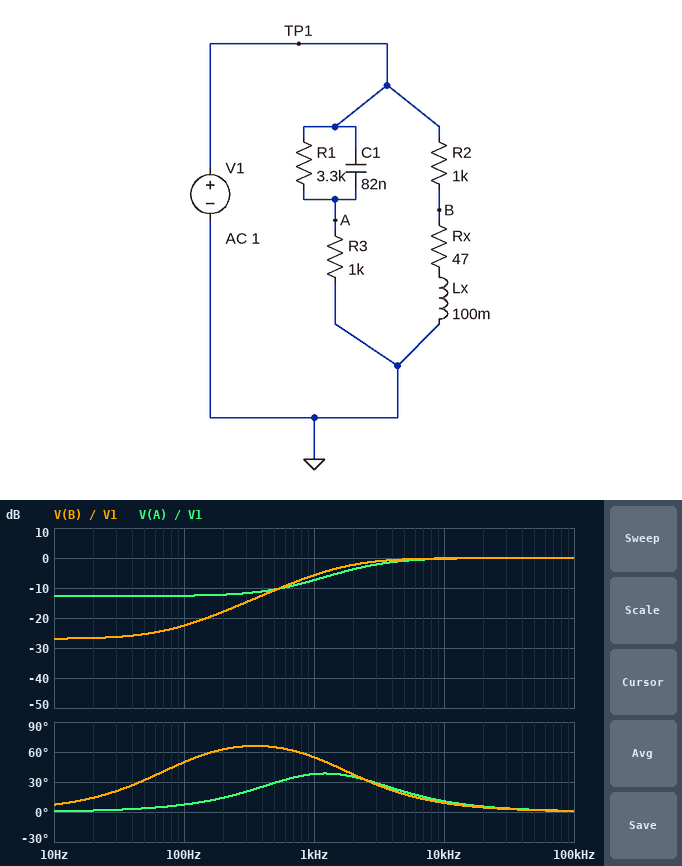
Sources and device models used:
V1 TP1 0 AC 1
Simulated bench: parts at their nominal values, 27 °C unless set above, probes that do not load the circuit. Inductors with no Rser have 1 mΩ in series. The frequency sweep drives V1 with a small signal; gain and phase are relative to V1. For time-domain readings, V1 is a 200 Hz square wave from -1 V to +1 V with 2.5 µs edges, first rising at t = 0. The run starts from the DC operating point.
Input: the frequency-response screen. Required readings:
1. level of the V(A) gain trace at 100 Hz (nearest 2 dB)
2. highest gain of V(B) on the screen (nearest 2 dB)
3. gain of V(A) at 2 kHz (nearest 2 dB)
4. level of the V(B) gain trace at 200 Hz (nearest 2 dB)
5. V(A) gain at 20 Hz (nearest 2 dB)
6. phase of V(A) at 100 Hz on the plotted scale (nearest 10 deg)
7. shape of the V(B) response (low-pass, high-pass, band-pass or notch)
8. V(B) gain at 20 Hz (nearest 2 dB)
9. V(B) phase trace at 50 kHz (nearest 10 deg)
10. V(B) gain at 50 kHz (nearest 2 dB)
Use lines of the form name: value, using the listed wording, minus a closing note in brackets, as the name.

level of the V(A) gain trace at 100 Hz: -12 dB
highest gain of V(B) on the screen: 0 dB
gain of V(A) at 2 kHz: -4 dB
level of the V(B) gain trace at 200 Hz: -18 dB
V(A) gain at 20 Hz: -12 dB
phase of V(A) at 100 Hz on the plotted scale: 10 deg
shape of the V(B) response: high-pass
V(B) gain at 20 Hz: -26 dB
V(B) phase trace at 50 kHz: 0 deg
V(B) gain at 50 kHz: 0 dB
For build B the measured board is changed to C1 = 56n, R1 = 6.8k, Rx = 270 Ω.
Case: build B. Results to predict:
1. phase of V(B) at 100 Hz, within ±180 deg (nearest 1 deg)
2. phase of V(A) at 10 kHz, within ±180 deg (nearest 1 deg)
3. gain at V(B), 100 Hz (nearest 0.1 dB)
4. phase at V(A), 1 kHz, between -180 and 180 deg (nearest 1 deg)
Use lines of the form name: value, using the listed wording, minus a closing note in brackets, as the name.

phase of V(B) at 100 Hz, within ±180 deg: 10 deg
phase of V(A) at 10 kHz, within ±180 deg: 16 deg
gain at V(B), 100 Hz: -13.2 dB
phase at V(A), 1 kHz, between -180 and 180 deg: 50 deg
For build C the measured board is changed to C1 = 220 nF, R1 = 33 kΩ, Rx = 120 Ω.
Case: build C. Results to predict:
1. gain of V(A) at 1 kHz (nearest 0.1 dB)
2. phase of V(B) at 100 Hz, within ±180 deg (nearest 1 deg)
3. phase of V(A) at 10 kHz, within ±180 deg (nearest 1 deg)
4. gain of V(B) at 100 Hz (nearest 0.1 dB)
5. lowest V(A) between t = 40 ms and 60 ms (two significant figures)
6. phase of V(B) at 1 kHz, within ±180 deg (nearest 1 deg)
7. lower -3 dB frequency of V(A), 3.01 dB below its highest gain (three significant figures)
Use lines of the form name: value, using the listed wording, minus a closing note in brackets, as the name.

gain of V(A) at 1 kHz: -1.9 dB
phase of V(B) at 100 Hz, within ±180 deg: 24 deg
phase of V(A) at 10 kHz, within ±180 deg: 4 deg
gain of V(B) at 100 Hz: -18.4 dB
lowest V(A) between t = 40 ms and 60 ms: -2.0 V
phase of V(B) at 1 kHz, within ±180 deg: 50 deg
lower -3 dB frequency of V(A), 3.01 dB below its highest gain: 745 Hz
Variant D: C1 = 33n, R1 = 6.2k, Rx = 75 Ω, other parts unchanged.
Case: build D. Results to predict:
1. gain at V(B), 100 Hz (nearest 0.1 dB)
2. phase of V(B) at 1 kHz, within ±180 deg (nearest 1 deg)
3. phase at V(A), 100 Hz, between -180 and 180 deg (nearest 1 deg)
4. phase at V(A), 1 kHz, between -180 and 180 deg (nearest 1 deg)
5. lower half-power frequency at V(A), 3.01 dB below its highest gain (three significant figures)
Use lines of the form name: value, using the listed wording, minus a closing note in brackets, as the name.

gain at V(B), 100 Hz: -20.8 dB
phase of V(B) at 1 kHz, within ±180 deg: 53 deg
phase at V(A), 100 Hz, between -180 and 180 deg: 6 deg
phase at V(A), 1 kHz, between -180 and 180 deg: 42 deg
lower half-power frequency at V(A), 3.01 dB below its highest gain: 5.49 kHz
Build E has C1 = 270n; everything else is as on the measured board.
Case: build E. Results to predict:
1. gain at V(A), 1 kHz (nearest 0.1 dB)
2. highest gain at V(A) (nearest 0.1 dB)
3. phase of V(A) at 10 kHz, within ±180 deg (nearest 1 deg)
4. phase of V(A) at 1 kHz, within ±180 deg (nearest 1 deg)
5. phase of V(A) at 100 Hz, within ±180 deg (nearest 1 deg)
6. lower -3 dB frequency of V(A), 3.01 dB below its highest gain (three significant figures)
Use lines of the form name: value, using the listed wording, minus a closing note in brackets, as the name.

gain at V(A), 1 kHz: -1.9 dB
highest gain at V(A): 0 dB
phase of V(A) at 10 kHz, within ±180 deg: 3 deg
phase of V(A) at 1 kHz, within ±180 deg: 27 deg
phase of V(A) at 100 Hz, within ±180 deg: 22 deg
lower -3 dB frequency of V(A), 3.01 dB below its highest gain: 725 Hz
